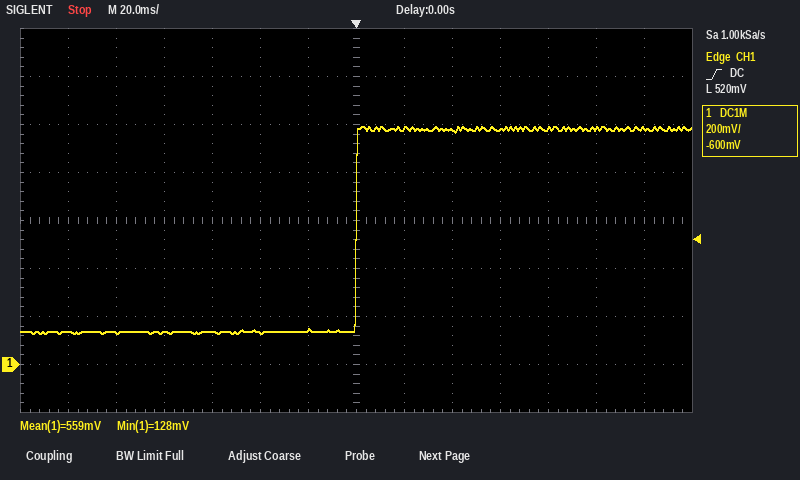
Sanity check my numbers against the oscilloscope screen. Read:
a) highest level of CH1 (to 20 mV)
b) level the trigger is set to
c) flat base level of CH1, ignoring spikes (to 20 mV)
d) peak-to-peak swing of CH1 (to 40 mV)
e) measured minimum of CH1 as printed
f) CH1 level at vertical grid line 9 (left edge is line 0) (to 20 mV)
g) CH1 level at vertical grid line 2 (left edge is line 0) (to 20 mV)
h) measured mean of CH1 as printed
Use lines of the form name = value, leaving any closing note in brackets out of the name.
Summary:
highest level of CH1 = 1.00 V
level the trigger is set to = 520 mV
flat base level of CH1, ignoring spikes = 140 mV
peak-to-peak swing of CH1 = 880 mV
measured minimum of CH1 as printed = 128 mV
CH1 level at vertical grid line 9 (left edge is line 0) = 980 mV
CH1 level at vertical grid line 2 (left edge is line 0) = 140 mV
measured mean of CH1 as printed = 559 mV
